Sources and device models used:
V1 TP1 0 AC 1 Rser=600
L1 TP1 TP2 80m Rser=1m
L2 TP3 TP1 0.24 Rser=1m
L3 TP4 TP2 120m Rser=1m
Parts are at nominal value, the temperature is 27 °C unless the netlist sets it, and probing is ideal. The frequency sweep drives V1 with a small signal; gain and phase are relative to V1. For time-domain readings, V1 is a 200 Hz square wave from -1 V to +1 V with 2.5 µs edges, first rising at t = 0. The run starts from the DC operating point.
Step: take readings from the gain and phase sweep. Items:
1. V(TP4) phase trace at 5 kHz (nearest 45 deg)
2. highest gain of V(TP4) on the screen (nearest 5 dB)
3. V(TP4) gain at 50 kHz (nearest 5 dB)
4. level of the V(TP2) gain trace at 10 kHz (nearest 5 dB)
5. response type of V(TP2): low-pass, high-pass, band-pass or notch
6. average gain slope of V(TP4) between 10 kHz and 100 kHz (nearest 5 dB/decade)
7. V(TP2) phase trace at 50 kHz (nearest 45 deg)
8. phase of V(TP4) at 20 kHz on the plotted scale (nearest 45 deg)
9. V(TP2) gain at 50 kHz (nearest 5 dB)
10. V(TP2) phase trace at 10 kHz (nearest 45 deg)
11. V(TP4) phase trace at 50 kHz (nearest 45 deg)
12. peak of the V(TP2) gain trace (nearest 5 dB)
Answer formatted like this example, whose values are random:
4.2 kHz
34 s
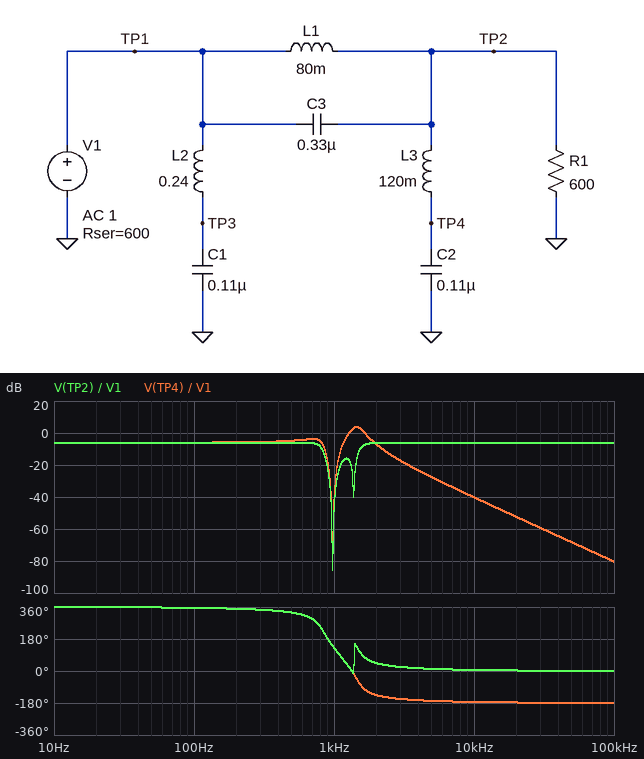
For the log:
-180 deg
5 dB
-70 dB
-5 dB
notch
-40 dB/decade
0 deg
-180 deg
-5 dB
0 deg
-180 deg
-5 dB
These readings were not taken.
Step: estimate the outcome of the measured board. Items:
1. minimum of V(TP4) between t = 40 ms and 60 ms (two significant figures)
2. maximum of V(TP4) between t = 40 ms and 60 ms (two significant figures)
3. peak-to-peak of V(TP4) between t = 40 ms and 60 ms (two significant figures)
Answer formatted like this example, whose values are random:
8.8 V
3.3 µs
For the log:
-990 mV
990 mV
2.0 V
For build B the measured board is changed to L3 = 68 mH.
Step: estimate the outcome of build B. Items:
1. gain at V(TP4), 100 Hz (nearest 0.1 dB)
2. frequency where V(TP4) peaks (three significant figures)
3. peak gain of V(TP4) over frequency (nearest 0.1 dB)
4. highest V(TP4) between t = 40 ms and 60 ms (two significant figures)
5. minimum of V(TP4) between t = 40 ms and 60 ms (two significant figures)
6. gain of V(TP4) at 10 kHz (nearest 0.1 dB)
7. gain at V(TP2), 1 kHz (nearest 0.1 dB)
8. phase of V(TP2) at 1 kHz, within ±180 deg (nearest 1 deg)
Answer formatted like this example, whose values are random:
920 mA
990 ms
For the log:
-6.0 dB
1.84 kHz
2.2 dB
980 mV
-980 mV
-35.1 dB
-47.3 dB
142 deg
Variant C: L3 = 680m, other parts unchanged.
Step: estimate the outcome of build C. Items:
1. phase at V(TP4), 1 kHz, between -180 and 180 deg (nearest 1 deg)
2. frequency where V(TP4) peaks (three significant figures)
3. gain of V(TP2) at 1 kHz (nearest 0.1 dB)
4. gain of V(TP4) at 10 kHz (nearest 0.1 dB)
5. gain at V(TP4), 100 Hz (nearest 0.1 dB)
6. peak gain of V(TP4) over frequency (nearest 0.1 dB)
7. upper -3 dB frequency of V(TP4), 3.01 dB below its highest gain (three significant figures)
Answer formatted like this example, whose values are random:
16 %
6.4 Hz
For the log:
3 deg
572 Hz
-45.9 dB
-55.4 dB
-5.8 dB
12.4 dB
604 Hz
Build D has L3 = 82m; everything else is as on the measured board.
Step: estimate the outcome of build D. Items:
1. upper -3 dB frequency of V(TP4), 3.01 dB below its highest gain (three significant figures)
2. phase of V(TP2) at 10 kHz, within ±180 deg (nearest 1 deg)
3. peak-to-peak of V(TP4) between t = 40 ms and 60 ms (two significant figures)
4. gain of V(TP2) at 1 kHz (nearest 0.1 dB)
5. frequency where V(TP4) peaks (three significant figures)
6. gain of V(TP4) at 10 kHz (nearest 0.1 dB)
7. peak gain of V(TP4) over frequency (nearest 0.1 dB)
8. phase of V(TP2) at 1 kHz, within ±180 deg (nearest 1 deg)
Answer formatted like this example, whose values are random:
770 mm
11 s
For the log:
1.96 kHz
7 deg
2.0 V
-47.5 dB
1.70 kHz
-36.8 dB
2.9 dB
139 deg
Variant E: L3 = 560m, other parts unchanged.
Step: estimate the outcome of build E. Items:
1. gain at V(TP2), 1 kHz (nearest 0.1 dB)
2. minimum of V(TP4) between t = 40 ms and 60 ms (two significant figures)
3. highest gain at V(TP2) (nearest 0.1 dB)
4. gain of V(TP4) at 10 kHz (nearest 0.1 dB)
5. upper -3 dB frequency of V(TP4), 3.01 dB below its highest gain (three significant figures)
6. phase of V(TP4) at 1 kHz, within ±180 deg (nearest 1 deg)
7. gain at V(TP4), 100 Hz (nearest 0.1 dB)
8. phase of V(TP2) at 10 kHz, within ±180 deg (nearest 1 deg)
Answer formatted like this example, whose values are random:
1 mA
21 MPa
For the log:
-46.0 dB
-1.9 V
-6.0 dB
-53.7 dB
662 Hz
8 deg
-5.8 dB
4 deg
